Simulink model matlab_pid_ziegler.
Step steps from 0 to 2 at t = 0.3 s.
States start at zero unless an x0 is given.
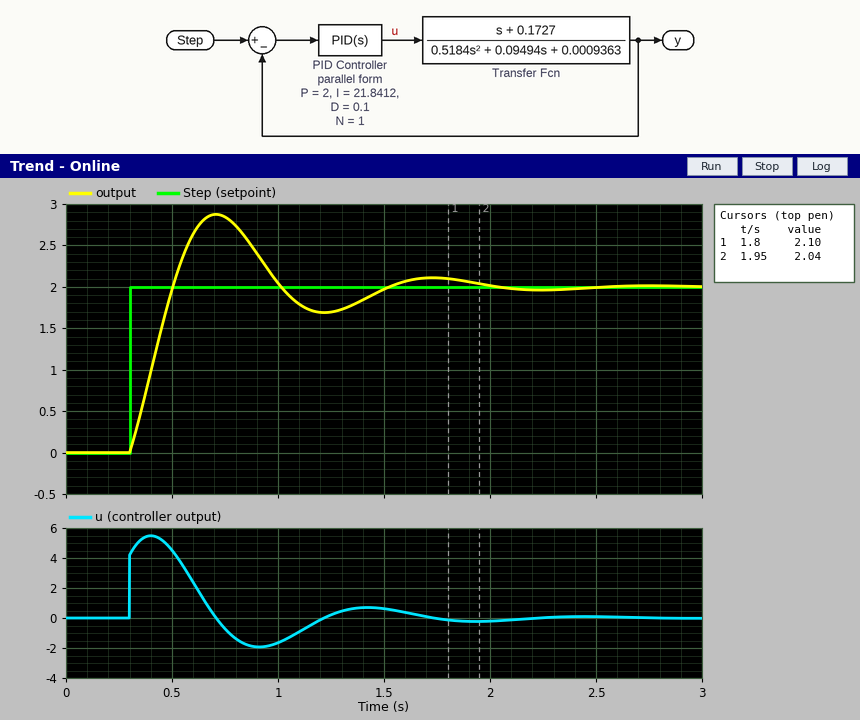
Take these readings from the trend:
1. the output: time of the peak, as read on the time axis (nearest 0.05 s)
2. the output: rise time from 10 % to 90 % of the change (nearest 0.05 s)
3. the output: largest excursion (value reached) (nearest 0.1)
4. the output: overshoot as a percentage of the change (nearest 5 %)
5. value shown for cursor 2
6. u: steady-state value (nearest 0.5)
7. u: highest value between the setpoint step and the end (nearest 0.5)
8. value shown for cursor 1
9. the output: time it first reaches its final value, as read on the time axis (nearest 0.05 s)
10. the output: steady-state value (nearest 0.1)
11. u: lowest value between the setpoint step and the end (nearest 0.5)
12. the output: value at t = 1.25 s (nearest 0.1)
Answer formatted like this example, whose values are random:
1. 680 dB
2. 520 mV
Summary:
1. 0.70 s
2. 0.15 s
3. 2.9
4. 45 %
5. 2.04
6. 0.0
7. 5.5
8. 2.10
9. 0.50 s
10. 2.0
11. -2.0
12. 1.7
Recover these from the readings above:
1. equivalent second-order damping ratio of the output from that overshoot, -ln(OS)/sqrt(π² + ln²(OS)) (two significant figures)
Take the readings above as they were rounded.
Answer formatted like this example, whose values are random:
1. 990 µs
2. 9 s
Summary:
1. 0.25
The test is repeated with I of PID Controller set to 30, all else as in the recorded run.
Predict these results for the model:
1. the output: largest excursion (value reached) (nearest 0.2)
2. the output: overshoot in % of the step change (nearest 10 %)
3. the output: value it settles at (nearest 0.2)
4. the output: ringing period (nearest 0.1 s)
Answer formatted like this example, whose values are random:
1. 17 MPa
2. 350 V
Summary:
1. 3.0
2. 50 %
3. 2.0
4. 0.9 s
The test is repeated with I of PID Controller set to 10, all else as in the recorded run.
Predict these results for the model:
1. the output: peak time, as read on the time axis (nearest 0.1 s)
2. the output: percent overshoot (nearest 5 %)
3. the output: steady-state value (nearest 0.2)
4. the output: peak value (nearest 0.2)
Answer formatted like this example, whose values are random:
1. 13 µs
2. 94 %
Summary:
1. 0.9 s
2. 30 %
3. 2.0
4. 2.6
